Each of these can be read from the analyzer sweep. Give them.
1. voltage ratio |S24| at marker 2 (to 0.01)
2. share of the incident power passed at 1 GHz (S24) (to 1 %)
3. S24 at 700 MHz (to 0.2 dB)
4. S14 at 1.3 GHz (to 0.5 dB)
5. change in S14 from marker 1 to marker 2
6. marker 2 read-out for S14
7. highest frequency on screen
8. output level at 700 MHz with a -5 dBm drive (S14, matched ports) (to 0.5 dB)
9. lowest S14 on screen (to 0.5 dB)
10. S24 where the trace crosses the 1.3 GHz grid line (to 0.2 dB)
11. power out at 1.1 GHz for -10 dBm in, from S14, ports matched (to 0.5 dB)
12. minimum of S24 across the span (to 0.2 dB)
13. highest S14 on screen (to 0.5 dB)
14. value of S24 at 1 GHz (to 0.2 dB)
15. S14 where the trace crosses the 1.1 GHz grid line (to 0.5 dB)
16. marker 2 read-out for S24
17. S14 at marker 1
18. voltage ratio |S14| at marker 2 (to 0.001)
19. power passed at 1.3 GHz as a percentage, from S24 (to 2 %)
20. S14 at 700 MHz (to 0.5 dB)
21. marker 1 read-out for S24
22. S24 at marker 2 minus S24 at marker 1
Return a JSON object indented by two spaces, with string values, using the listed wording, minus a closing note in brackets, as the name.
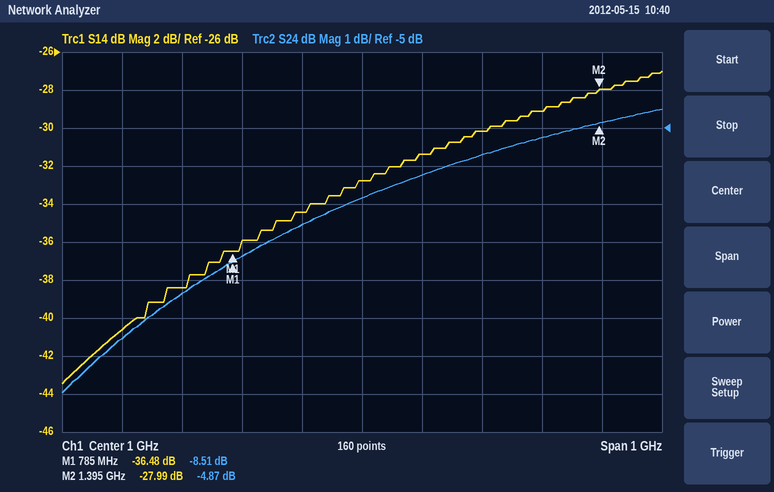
{
  "voltage ratio |S24| at marker 2": "0.57",
  "share of the incident power passed at 1 GHz (S24)": "21 %",
  "S24 at 700 MHz": "-9.4 dB",
  "S14 at 1.3 GHz": "-29.0 dB",
  "change in S14 from marker 1 to marker 2": "8.49 dB",
  "marker 2 read-out for S14": "-27.99 dB",
  "highest frequency on screen": "1.5 GHz",
  "output level at 700 MHz with a -5 dBm drive (S14, matched ports)": "-43.5 dBm",
  "lowest S14 on screen": "-43.5 dB",
  "S24 where the trace crosses the 1.3 GHz grid line": "-5.2 dB",
  "power out at 1.1 GHz for -10 dBm in, from S14, ports matched": "-41.5 dBm",
  "minimum of S24 across the span": "-12.0 dB",
  "highest S14 on screen": "-27.0 dB",
  "value of S24 at 1 GHz": "-6.8 dB",
  "S14 where the trace crosses the 1.1 GHz grid line": "-31.5 dB",
  "marker 2 read-out for S24": "-4.87 dB",
  "S14 at marker 1": "-36.48 dB",
  "voltage ratio |S14| at marker 2": "0.040",
  "power passed at 1.3 GHz as a percentage, from S24": "30 %",
  "S14 at 700 MHz": "-38.5 dB",
  "marker 1 read-out for S24": "-8.51 dB",
  "S24 at marker 2 minus S24 at marker 1": "3.64 dB"
}
